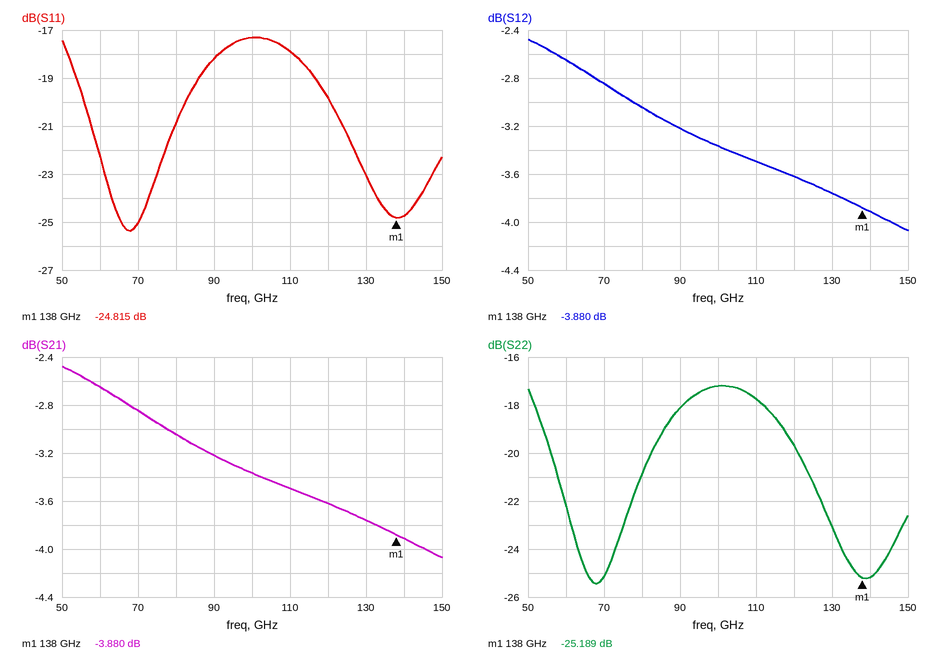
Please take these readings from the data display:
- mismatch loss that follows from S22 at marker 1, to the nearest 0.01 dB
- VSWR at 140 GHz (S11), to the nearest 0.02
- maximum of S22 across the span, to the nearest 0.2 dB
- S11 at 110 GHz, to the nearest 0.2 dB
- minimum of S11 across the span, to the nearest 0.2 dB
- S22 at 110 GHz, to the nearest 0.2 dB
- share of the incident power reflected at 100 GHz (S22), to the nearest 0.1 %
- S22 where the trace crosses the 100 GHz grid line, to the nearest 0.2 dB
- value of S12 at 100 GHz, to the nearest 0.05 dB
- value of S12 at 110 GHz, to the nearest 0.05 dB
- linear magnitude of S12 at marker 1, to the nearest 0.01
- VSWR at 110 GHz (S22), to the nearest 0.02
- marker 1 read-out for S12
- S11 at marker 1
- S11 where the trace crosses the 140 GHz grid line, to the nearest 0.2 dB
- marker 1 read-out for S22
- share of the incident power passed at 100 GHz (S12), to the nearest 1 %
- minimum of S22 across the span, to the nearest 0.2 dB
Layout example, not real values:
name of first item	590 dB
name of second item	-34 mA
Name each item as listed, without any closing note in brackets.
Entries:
mismatch loss that follows from S22 at marker 1, to the nearest 0.01 dB	0.01 dB
VSWR at 140 GHz (S11), to the nearest 0.02	1.12
maximum of S22 across the span, to the nearest 0.2 dB	-17.2 dB
S11 at 110 GHz, to the nearest 0.2 dB	-17.8 dB
minimum of S11 across the span, to the nearest 0.2 dB	-25.4 dB
S22 at 110 GHz, to the nearest 0.2 dB	-17.8 dB
share of the incident power reflected at 100 GHz (S22), to the nearest 0.1 %	1.9 %
S22 where the trace crosses the 100 GHz grid line, to the nearest 0.2 dB	-17.2 dB
value of S12 at 100 GHz, to the nearest 0.05 dB	-3.35 dB
value of S12 at 110 GHz, to the nearest 0.05 dB	-3.50 dB
linear magnitude of S12 at marker 1, to the nearest 0.01	0.64
VSWR at 110 GHz (S22), to the nearest 0.02	1.30
marker 1 read-out for S12	-3.880 dB
S11 at marker 1	-24.815 dB
S11 where the trace crosses the 140 GHz grid line, to the nearest 0.2 dB	-24.8 dB
marker 1 read-out for S22	-25.189 dB
share of the incident power passed at 100 GHz (S12), to the nearest 1 %	46 %
minimum of S22 across the span, to the nearest 0.2 dB	-25.4 dB
